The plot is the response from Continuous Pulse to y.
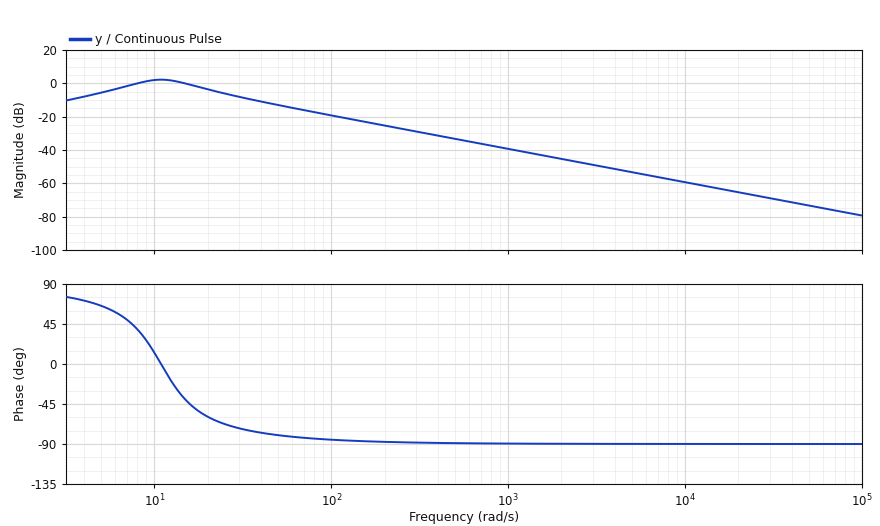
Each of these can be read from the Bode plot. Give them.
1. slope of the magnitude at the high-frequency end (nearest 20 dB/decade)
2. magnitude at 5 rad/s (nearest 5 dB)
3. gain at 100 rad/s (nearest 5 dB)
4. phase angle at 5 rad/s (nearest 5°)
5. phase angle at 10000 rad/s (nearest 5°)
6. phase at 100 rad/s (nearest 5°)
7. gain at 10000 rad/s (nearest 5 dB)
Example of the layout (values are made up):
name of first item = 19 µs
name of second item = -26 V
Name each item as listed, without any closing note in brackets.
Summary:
slope of the magnitude at the high-frequency end = -20 dB/decade
magnitude at 5 rad/s = -5 dB
gain at 100 rad/s = -20 dB
phase angle at 5 rad/s = 65°
phase angle at 10000 rad/s = -90°
phase at 100 rad/s = -85°
gain at 10000 rad/s = -60 dB
